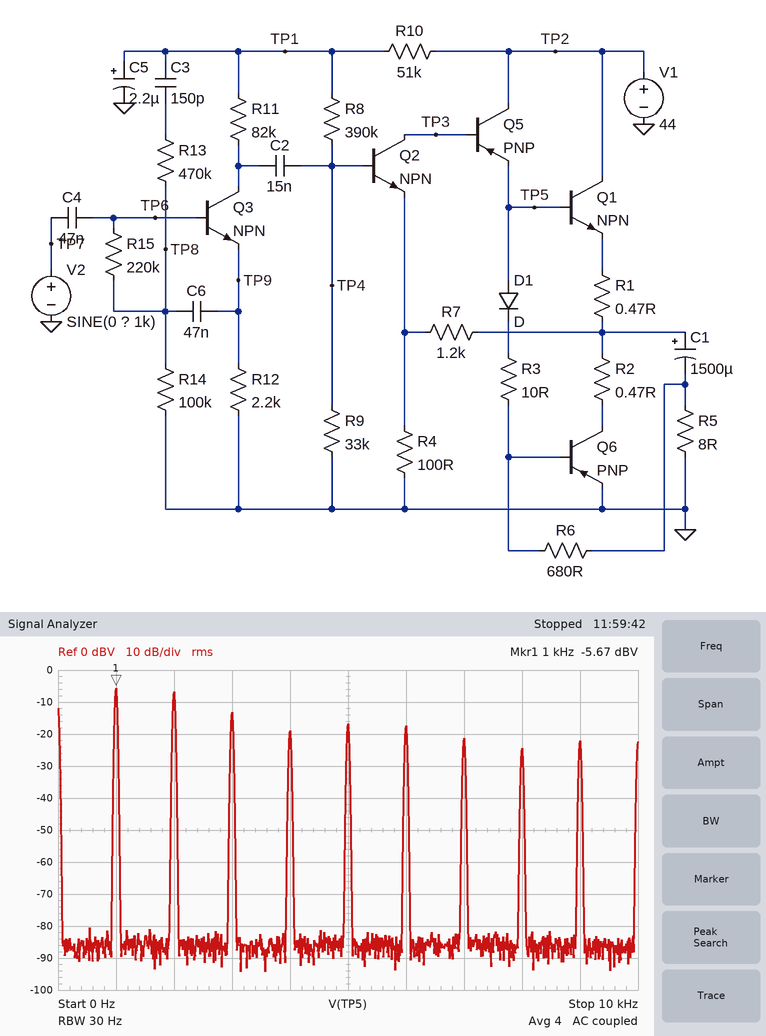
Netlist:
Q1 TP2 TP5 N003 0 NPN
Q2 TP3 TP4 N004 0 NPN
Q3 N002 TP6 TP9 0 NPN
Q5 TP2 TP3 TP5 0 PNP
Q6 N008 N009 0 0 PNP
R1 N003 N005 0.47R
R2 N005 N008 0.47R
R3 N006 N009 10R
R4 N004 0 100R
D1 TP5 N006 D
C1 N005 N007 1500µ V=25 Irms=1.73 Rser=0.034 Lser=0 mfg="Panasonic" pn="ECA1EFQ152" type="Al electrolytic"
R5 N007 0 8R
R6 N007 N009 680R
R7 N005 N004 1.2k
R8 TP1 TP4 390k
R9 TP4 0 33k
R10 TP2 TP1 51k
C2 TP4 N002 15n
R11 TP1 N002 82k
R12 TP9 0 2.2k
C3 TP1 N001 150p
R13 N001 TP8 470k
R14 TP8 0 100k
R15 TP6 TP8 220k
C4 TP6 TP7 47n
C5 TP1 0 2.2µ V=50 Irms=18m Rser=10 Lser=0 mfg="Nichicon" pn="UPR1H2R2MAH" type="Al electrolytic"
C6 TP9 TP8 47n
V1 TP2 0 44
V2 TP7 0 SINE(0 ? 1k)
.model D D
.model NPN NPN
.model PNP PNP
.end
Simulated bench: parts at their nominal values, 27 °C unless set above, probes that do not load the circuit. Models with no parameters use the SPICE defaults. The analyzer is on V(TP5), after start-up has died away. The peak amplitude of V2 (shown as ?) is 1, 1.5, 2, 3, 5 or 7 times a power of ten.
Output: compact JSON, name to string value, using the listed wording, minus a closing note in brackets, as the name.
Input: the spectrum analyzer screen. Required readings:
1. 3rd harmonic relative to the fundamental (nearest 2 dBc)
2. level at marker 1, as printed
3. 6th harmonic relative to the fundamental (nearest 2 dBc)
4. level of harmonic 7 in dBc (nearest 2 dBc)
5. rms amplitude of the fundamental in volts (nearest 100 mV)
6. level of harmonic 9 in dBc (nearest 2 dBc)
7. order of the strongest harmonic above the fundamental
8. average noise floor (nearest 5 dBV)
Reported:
{"3rd harmonic relative to the fundamental": "-8 dBc", "level at marker 1, as printed": "-5.67 dBV", "6th harmonic relative to the fundamental": "-12 dBc", "level of harmonic 7 in dBc": "-16 dBc", "rms amplitude of the fundamental in volts": "500 mV", "level of harmonic 9 in dBc": "-16 dBc", "order of the strongest harmonic above the fundamental": "2", "average noise floor": "-85 dBV"}
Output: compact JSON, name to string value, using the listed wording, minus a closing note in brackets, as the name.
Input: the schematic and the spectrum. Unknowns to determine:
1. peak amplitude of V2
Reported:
{"peak amplitude of V2": "7 V"}
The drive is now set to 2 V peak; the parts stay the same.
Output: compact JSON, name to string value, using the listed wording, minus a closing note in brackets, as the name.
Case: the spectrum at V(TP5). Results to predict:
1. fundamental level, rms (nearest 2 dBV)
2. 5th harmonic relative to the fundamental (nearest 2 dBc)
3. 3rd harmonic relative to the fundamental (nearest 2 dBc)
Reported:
{"fundamental level, rms": "-4 dBV", "5th harmonic relative to the fundamental": "-14 dBc", "3rd harmonic relative to the fundamental": "-12 dBc"}
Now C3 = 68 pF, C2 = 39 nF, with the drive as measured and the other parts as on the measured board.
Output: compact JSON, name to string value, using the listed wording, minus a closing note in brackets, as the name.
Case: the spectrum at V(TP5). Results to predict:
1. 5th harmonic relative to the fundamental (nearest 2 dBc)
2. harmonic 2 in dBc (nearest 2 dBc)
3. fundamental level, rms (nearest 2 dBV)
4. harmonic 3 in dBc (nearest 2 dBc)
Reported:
{"5th harmonic relative to the fundamental": "-14 dBc", "harmonic 2 in dBc": "-4 dBc", "fundamental level, rms": "-4 dBV", "harmonic 3 in dBc": "-10 dBc"}
